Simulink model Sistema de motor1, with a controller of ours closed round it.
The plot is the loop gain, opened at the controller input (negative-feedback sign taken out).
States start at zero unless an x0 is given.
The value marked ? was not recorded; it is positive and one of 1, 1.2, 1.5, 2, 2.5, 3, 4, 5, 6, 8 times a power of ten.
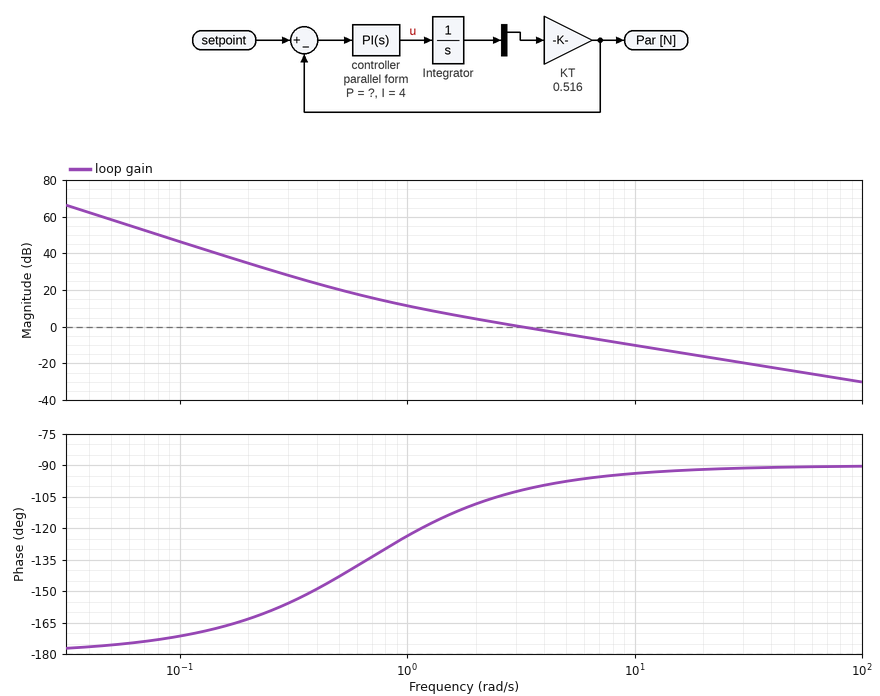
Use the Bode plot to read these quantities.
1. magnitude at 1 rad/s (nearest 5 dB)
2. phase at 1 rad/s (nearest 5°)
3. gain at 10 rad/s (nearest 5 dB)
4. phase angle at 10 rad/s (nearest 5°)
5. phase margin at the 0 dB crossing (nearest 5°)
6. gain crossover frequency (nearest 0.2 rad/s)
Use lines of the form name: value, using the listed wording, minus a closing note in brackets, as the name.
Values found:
magnitude at 1 rad/s: 10 dB
phase at 1 rad/s: -125°
gain at 10 rad/s: -10 dB
phase angle at 10 rad/s: -95°
phase margin at the 0 dB crossing: 80°
gain crossover frequency: 3.2 rad/s
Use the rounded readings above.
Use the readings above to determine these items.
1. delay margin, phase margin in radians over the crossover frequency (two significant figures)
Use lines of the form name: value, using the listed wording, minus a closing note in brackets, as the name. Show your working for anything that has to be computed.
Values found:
delay margin, phase margin in radians over the crossover frequency: 80 × π / 180 / 3.2 = 0.44 s
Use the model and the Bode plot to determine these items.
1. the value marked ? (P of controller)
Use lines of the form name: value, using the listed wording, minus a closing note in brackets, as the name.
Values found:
the value marked ?: 6
